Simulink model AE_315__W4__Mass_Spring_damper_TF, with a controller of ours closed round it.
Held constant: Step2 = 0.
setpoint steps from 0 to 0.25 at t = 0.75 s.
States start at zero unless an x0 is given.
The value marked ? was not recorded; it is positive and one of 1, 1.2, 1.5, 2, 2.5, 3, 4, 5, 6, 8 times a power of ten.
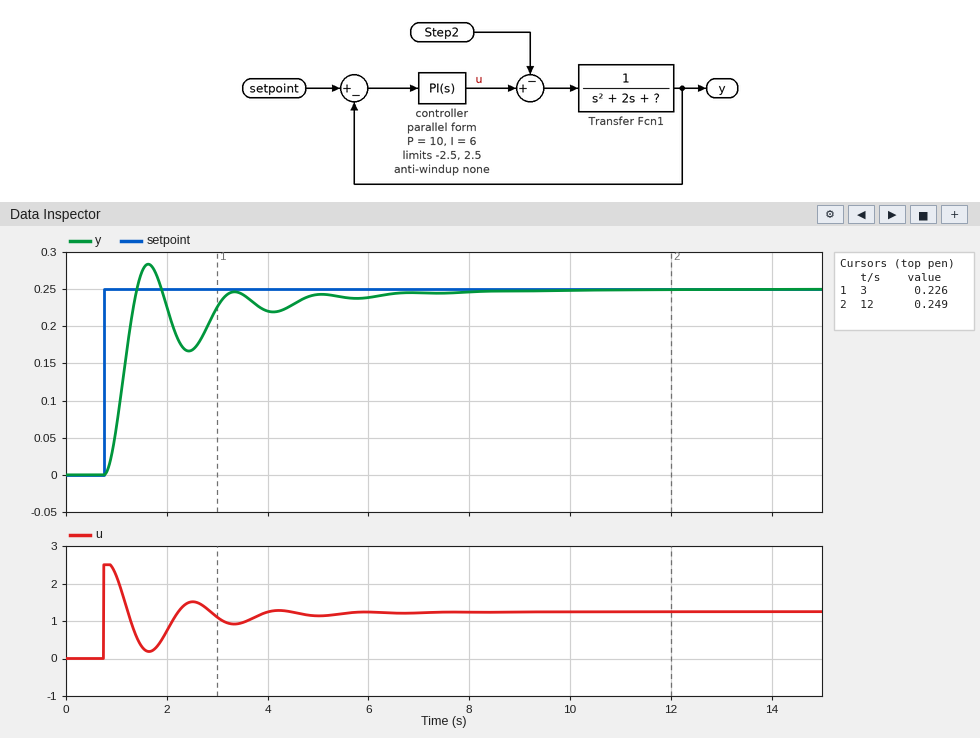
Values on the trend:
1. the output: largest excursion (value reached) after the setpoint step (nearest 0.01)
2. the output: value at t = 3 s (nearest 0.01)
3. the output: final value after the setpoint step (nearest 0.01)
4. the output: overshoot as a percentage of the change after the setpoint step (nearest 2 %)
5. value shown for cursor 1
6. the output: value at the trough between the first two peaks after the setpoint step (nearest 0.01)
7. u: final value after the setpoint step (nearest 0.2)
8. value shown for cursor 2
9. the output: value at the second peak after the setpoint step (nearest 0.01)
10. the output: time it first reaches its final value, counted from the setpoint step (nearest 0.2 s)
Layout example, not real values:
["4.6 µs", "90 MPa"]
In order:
["0.28", "0.23", "0.25", "14 %", "0.226", "0.17", "1.2", "0.249", "0.25", "0.6 s"]
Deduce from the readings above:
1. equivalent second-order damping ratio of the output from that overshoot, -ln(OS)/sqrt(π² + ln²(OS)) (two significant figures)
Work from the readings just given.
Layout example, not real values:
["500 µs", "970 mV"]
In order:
["0.53"]
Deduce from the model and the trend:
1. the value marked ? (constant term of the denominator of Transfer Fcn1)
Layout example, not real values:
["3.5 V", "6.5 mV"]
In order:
["5"]
